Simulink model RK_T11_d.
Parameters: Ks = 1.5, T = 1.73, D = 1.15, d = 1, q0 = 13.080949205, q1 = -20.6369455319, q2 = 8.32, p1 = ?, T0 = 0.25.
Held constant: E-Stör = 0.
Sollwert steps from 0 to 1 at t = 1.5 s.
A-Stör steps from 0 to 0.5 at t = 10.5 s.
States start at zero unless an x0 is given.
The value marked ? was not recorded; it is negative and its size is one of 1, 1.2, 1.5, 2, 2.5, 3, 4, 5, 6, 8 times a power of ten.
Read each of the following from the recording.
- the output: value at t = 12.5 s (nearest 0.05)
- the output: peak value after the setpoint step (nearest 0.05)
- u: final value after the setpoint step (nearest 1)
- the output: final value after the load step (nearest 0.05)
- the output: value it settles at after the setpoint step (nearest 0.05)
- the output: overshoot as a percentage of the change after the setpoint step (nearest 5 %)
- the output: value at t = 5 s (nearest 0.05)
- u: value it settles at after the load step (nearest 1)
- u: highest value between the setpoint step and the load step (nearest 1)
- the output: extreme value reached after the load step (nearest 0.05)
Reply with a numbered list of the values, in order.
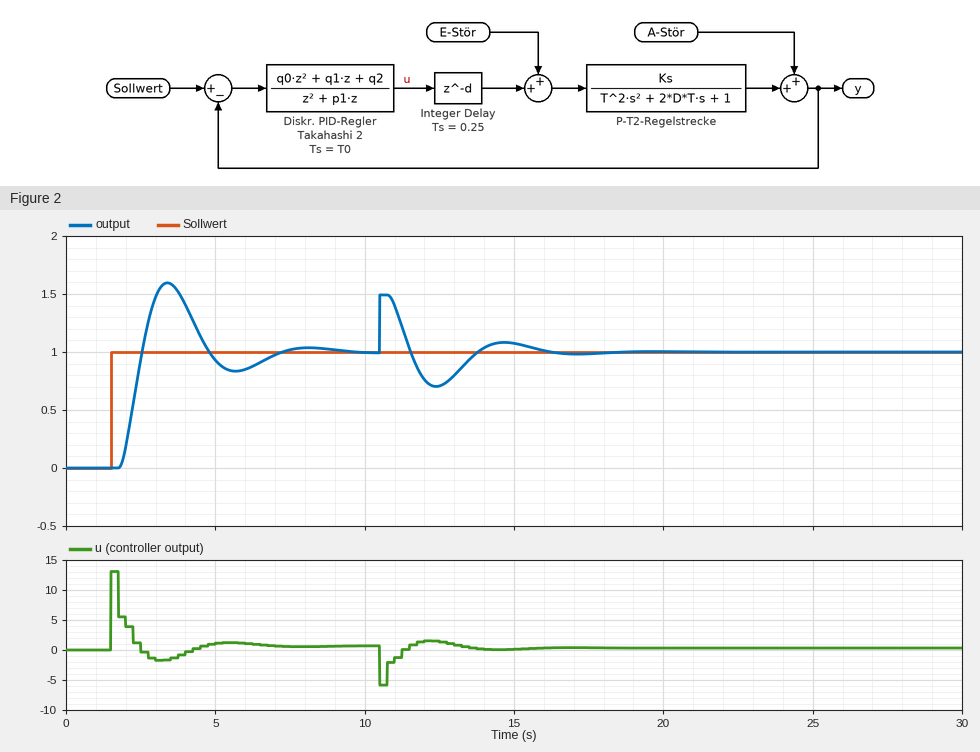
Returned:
1. 0.70
2. 1.60
3. 1
4. 1.00
5. 1.00
6. 60 %
7. 0.95
8. 0
9. 13
10. 1.50
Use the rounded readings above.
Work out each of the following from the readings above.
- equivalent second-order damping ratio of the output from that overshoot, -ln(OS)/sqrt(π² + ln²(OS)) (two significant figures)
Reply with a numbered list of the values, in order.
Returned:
1. 0.16
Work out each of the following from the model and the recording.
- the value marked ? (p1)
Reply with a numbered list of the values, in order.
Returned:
1. -1
